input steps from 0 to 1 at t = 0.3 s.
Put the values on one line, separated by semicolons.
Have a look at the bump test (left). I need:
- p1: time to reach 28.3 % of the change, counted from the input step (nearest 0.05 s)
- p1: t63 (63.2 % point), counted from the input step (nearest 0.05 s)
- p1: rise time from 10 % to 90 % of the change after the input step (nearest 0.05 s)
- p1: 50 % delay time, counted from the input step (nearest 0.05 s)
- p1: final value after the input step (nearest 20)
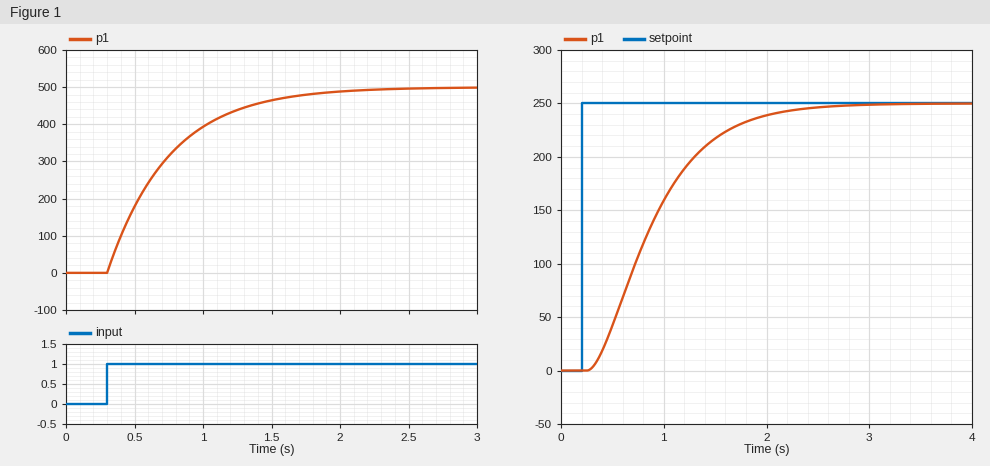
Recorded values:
0.15 s; 0.45 s; 1.00 s; 0.30 s; 500
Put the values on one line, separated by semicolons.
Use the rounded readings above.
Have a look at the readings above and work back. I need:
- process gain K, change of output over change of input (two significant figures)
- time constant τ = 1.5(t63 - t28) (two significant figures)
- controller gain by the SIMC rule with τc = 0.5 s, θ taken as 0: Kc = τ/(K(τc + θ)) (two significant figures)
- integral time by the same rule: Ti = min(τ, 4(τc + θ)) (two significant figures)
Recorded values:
500; 0.45 s; 0.0018; 0.45 s
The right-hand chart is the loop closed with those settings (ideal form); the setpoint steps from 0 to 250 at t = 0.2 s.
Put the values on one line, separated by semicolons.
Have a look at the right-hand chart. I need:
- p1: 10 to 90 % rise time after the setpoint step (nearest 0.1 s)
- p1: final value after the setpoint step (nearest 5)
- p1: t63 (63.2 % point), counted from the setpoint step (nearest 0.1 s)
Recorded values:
1.2 s; 250; 0.8 s
